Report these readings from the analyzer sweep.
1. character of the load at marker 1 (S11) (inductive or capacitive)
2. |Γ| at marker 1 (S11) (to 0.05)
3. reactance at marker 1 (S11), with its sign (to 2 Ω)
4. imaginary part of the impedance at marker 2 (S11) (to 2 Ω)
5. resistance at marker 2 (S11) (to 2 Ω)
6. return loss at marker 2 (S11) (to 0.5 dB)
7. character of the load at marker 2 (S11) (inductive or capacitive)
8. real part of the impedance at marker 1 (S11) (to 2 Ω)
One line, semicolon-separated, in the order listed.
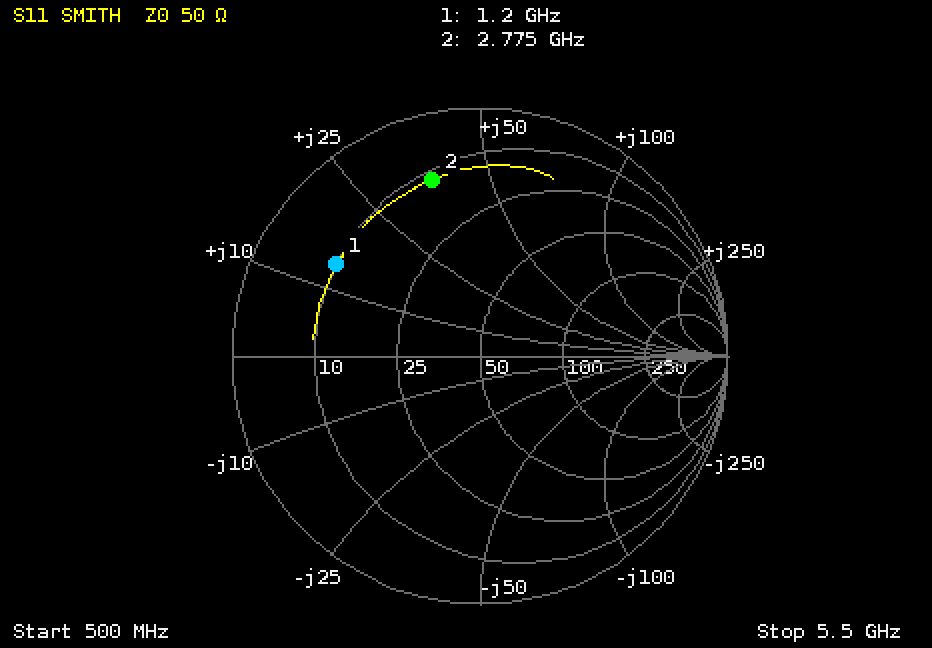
inductive; 0.70; +14 Ω; +36 Ω; 12 Ω; 2.5 dB; inductive; 10 Ω
